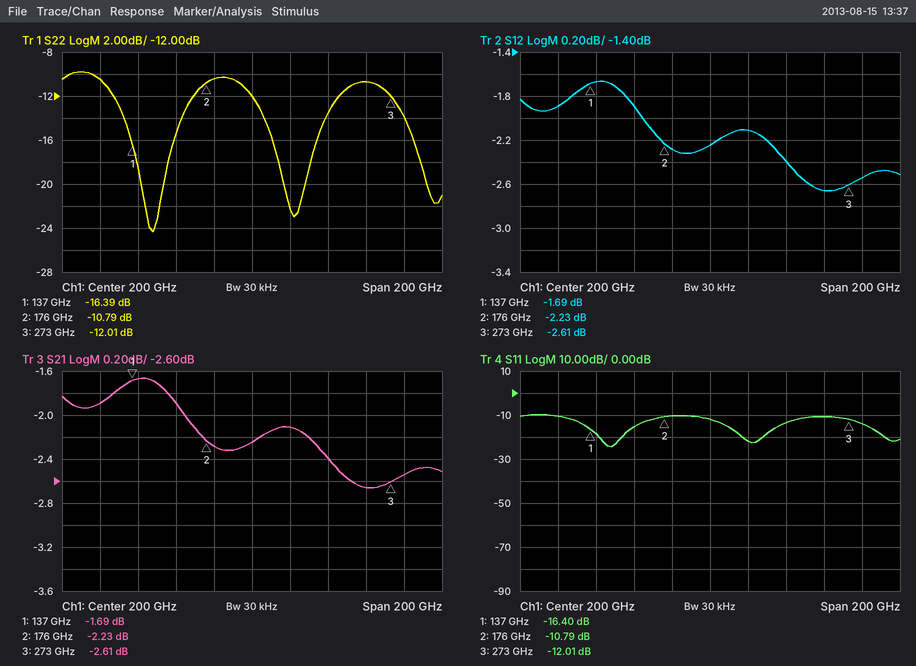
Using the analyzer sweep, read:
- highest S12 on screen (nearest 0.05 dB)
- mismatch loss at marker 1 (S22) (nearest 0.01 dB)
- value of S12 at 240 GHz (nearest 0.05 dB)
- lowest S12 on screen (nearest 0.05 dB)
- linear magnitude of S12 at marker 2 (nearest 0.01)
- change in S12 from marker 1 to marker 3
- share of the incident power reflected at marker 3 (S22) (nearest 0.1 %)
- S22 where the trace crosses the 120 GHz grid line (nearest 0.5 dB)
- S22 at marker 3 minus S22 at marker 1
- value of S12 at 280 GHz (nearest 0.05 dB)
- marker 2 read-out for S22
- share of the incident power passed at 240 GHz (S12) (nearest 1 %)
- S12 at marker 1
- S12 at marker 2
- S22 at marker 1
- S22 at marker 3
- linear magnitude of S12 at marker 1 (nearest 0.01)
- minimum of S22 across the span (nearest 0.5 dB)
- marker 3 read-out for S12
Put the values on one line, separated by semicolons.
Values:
-1.65 dB; 0.10 dB; -2.40 dB; -2.65 dB; 0.77; -0.92 dB; 6.3 %; -10.5 dB; 4.38 dB; -2.55 dB; -10.79 dB; 58 %; -1.69 dB; -2.23 dB; -16.39 dB; -12.01 dB; 0.82; -24.5 dB; -2.61 dB
